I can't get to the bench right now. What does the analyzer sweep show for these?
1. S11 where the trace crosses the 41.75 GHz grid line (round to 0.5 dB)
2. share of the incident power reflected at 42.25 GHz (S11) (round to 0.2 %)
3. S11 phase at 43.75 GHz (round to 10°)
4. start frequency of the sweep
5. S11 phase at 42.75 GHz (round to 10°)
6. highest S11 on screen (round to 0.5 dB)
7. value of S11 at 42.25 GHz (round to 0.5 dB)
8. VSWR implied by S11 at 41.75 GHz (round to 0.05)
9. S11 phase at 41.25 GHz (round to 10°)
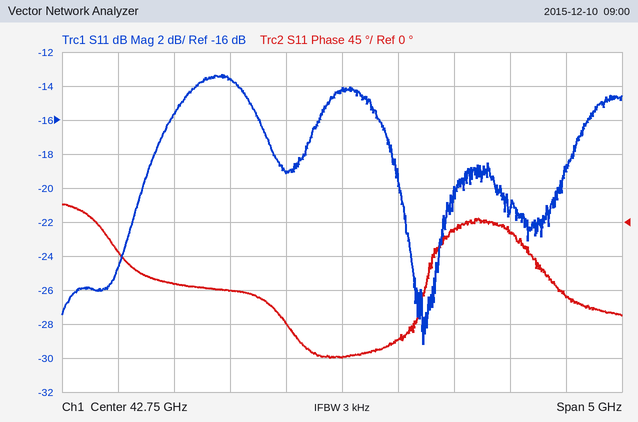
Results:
-13.5 dB
1.2 %
-10°
40.25 GHz
-180°
-13.5 dB
-19.0 dB
1.55
-80°
